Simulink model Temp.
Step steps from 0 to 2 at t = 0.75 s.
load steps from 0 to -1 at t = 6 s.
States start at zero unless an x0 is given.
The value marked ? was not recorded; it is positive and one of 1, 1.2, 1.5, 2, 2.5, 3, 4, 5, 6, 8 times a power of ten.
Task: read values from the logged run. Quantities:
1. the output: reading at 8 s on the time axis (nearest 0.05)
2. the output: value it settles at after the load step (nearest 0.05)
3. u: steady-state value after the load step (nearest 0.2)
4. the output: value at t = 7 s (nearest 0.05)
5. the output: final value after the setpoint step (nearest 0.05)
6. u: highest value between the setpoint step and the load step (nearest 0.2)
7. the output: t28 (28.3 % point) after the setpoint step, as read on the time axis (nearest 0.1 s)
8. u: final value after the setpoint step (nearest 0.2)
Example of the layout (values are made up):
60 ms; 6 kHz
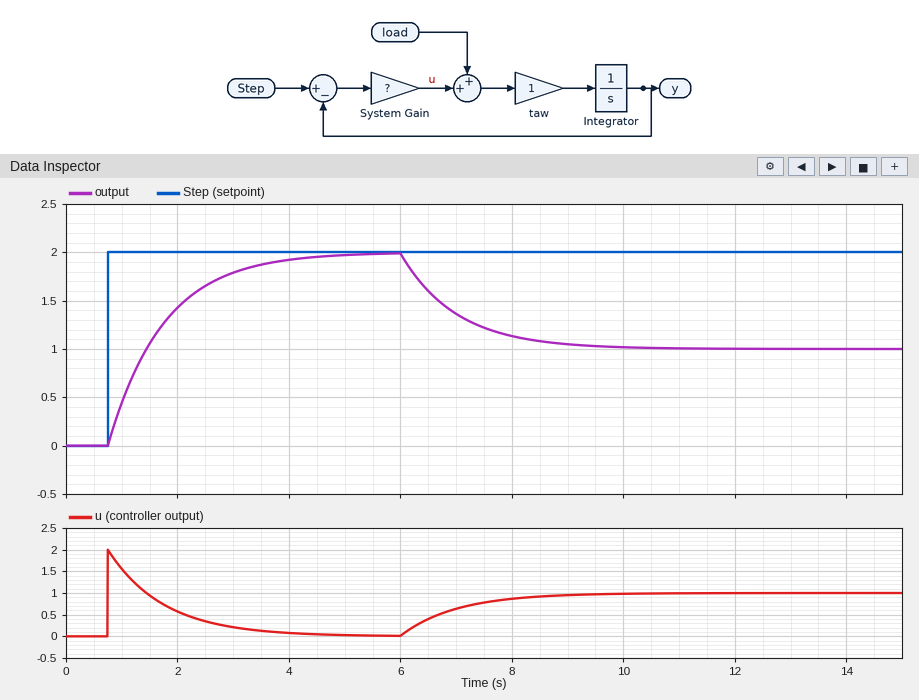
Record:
1.15; 1.00; 1.0; 1.35; 2.00; 2.0; 1.1 s; 0.0
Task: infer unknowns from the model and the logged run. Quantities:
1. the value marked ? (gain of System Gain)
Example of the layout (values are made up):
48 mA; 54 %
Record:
1
